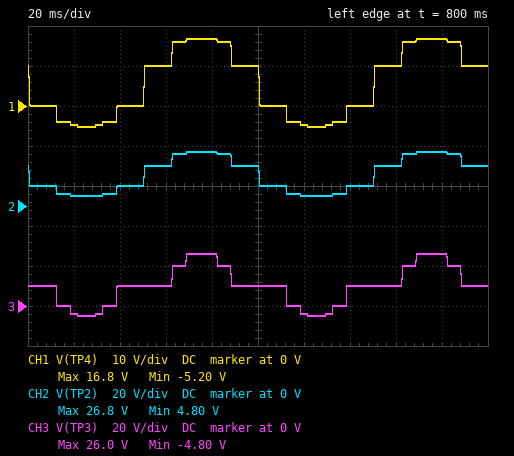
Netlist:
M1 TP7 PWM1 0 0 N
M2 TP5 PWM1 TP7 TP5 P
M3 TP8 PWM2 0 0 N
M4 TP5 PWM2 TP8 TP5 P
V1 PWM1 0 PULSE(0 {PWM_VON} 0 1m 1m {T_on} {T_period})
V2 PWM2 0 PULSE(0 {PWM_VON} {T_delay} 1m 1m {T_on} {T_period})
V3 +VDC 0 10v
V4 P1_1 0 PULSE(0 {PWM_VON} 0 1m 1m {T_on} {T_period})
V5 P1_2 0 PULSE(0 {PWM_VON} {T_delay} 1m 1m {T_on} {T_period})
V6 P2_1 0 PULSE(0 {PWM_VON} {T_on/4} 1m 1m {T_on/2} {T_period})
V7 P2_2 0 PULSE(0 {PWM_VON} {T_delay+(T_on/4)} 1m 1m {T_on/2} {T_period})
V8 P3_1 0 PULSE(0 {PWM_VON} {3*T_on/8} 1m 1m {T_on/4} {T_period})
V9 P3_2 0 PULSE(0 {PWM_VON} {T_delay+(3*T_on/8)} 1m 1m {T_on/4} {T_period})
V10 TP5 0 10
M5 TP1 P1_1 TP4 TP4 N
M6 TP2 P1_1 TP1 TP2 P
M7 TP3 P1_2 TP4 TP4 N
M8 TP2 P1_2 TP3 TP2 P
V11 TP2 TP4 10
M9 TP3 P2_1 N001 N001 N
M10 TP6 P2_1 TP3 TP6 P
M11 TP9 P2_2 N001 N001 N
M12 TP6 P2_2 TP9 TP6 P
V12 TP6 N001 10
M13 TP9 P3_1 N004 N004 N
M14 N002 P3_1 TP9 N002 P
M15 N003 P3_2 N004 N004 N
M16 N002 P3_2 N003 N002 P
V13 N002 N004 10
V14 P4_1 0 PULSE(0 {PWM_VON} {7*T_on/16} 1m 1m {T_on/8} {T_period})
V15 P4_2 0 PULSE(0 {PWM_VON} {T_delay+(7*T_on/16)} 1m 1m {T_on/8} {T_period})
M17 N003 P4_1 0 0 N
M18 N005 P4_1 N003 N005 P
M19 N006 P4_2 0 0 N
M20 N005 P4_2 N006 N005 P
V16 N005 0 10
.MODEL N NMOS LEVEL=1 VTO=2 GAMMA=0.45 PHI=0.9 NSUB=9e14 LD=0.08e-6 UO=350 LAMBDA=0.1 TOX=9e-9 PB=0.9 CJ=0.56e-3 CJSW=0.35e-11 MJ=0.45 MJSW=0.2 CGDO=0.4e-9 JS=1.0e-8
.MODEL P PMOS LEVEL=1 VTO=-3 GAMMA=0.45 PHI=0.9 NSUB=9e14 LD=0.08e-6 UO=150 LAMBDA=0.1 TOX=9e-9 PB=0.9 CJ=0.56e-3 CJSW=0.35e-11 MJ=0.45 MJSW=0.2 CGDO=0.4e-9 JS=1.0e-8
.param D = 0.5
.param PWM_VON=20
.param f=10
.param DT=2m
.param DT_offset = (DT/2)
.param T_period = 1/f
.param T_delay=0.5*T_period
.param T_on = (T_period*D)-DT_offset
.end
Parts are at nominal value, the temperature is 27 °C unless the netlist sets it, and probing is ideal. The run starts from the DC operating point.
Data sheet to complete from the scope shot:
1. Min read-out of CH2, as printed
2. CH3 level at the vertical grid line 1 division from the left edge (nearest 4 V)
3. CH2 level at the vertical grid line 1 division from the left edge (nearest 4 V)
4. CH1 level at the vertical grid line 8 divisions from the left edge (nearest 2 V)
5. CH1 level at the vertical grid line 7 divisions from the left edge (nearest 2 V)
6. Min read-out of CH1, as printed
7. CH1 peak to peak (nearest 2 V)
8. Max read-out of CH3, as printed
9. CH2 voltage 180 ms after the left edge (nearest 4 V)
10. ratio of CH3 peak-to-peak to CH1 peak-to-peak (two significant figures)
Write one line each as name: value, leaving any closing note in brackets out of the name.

Min read-out of CH2, as printed: 4.80 V
CH3 level at the vertical grid line 1 division from the left edge: -4 V
CH2 level at the vertical grid line 1 division from the left edge: 4 V
CH1 level at the vertical grid line 8 divisions from the left edge: 10 V
CH1 level at the vertical grid line 7 divisions from the left edge: 0 V
Min read-out of CH1, as printed: -5.20 V
CH1 peak to peak: 22 V
Max read-out of CH3, as printed: 26.0 V
CH2 voltage 180 ms after the left edge: 28 V
ratio of CH3 peak-to-peak to CH1 peak-to-peak: 1.4
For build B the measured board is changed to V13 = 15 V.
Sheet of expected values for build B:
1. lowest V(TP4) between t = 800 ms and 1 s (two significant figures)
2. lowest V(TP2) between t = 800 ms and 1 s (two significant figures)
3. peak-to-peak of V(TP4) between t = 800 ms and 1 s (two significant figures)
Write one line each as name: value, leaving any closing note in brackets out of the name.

lowest V(TP4) between t = 800 ms and 1 s: -6.3 V
lowest V(TP2) between t = 800 ms and 1 s: 3.7 V
peak-to-peak of V(TP4) between t = 800 ms and 1 s: 23 V
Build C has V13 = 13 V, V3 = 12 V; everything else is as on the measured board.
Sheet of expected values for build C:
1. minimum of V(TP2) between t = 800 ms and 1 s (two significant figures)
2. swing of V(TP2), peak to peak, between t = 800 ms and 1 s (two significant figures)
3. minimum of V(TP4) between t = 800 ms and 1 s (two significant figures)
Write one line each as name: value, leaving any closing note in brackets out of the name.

minimum of V(TP2) between t = 800 ms and 1 s: 4.3 V
swing of V(TP2), peak to peak, between t = 800 ms and 1 s: 23 V
minimum of V(TP4) between t = 800 ms and 1 s: -5.7 V
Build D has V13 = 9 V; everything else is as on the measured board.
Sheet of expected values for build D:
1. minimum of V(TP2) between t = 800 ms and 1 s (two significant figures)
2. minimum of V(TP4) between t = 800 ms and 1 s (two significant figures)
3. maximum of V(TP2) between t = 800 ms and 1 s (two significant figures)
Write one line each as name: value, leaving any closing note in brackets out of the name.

minimum of V(TP2) between t = 800 ms and 1 s: 4.9 V
minimum of V(TP4) between t = 800 ms and 1 s: -5.1 V
maximum of V(TP2) between t = 800 ms and 1 s: 27 V
